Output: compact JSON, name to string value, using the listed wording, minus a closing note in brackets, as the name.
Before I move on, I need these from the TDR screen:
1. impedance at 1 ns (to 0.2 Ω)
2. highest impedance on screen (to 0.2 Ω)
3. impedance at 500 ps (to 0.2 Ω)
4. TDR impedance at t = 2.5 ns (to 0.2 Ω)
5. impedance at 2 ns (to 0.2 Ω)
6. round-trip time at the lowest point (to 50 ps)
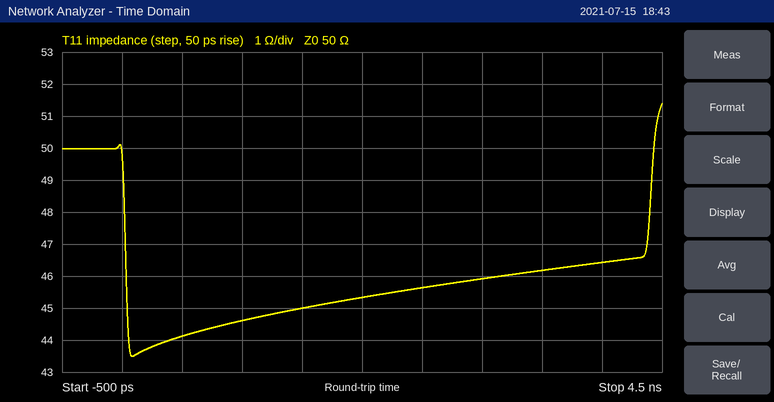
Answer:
{"impedance at 1 ns": "44.6 Ω", "highest impedance on screen": "51.4 Ω", "impedance at 500 ps": "44.2 Ω", "TDR impedance at t = 2.5 ns": "45.6 Ω", "impedance at 2 ns": "45.4 Ω", "round-trip time at the lowest point": "100 ps"}
